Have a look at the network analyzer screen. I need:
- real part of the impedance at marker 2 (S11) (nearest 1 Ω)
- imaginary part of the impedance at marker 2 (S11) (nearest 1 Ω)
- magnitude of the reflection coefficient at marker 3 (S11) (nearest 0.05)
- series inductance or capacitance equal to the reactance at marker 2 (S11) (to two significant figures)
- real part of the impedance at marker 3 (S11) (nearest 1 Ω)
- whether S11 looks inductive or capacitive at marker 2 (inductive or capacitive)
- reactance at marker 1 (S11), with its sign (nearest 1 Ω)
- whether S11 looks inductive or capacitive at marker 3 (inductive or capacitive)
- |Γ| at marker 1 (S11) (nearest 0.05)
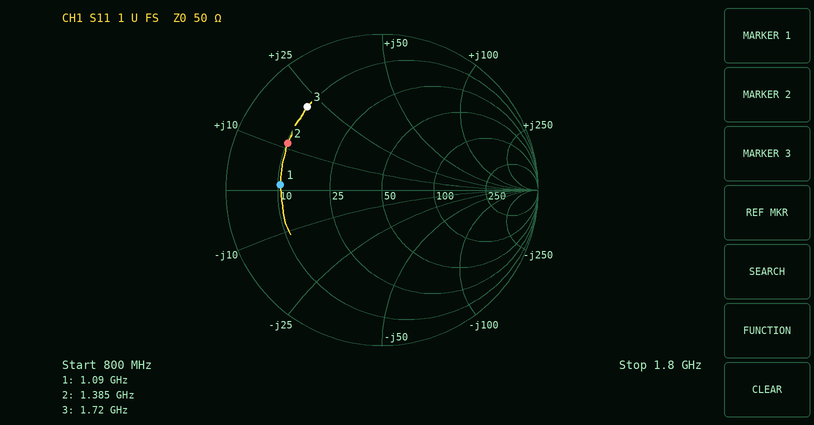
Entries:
10 Ω
+11 Ω
0.70
1.3 nH
10 Ω
inductive
+1 Ω
inductive
0.65
